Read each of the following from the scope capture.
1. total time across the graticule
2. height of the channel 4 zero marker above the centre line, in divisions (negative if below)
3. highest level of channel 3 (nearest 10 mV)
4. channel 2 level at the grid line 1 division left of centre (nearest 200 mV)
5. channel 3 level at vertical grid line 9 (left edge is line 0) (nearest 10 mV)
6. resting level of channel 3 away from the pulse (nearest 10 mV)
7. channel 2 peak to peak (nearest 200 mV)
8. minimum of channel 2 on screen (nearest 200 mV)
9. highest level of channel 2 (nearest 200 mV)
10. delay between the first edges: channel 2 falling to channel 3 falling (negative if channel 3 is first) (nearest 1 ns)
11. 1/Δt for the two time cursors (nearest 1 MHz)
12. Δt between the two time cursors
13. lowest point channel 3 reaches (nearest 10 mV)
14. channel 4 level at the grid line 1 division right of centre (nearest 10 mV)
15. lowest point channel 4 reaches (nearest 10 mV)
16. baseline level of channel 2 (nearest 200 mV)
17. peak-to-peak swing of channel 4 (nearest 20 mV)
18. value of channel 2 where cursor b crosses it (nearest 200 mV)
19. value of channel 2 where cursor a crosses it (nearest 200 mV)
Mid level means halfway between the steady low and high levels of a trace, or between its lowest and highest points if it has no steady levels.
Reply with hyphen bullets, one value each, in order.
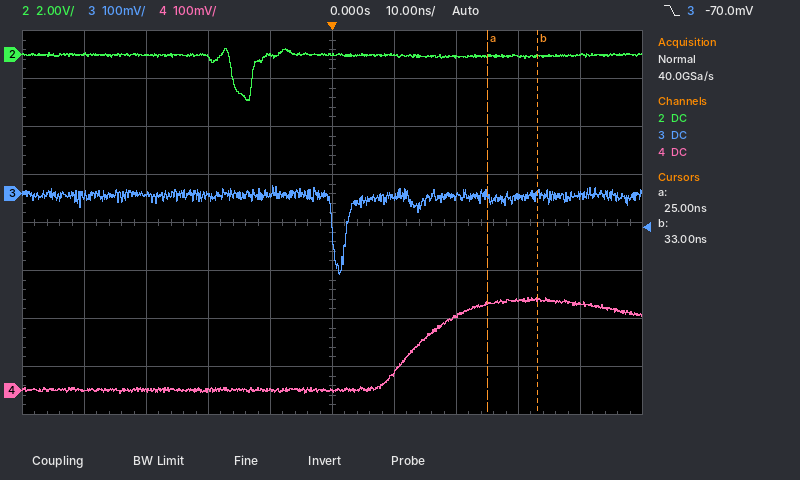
- 100 ns
- -3.5 div
- 20 mV
- 0.0 V
- 0 mV
- 0 mV
- 2.2 V
- -2.0 V
- 200 mV
- +16 ns
- 125 MHz
- 8 ns
- -170 mV
- 40 mV
- -10 mV
- 0.0 V
- 200 mV
- 0.0 V
- 0.0 V
